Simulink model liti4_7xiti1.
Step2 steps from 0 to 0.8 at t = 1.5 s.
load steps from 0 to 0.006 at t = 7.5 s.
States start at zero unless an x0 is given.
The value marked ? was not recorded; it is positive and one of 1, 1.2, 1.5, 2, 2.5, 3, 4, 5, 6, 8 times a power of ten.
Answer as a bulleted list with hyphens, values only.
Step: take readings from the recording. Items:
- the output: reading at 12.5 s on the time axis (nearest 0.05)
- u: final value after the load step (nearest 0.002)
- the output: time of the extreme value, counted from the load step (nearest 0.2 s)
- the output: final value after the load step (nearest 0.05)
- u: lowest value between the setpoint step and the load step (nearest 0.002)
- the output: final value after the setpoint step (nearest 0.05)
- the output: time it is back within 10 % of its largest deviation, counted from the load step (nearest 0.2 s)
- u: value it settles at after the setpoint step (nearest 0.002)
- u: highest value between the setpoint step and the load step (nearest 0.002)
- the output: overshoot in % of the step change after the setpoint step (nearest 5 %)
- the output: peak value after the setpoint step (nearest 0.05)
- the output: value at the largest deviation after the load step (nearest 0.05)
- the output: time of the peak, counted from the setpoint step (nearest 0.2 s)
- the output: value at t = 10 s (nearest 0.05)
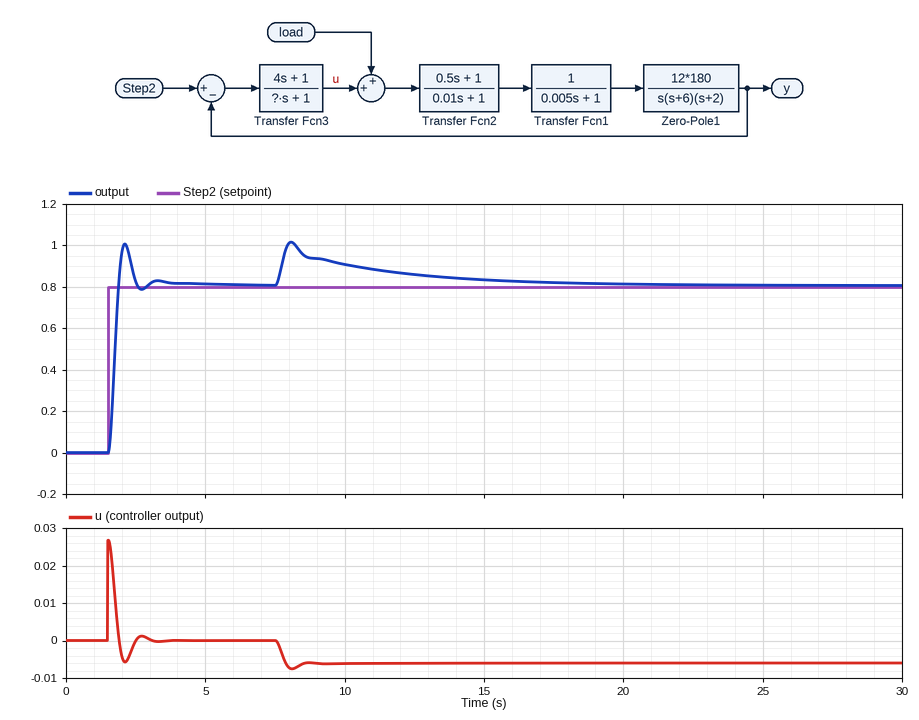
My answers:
- 0.85
- -0.006
- 0.6 s
- 0.80
- -0.006
- 0.80
- 8.6 s
- 0.000
- 0.026
- 25 %
- 1.00
- 1.00
- 0.6 s
- 0.90
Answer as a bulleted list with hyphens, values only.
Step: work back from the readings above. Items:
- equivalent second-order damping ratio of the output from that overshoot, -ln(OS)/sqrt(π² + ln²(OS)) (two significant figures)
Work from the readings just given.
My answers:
- 0.40
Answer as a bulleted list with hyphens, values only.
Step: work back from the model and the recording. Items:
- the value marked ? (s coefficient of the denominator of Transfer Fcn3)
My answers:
- 120
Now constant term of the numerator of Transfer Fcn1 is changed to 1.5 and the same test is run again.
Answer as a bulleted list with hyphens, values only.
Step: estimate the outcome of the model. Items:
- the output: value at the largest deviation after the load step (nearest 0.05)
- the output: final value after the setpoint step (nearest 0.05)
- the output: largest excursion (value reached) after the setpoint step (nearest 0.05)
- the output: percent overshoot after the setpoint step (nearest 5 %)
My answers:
- 1.05
- 0.80
- 1.10
- 35 %
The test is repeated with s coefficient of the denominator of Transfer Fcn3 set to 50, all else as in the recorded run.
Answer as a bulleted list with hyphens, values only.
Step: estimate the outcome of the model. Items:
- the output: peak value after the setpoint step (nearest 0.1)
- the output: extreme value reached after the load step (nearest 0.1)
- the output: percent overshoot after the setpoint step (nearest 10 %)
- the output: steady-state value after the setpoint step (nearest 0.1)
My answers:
- 1.2
- 0.9
- 50 %
- 0.8
